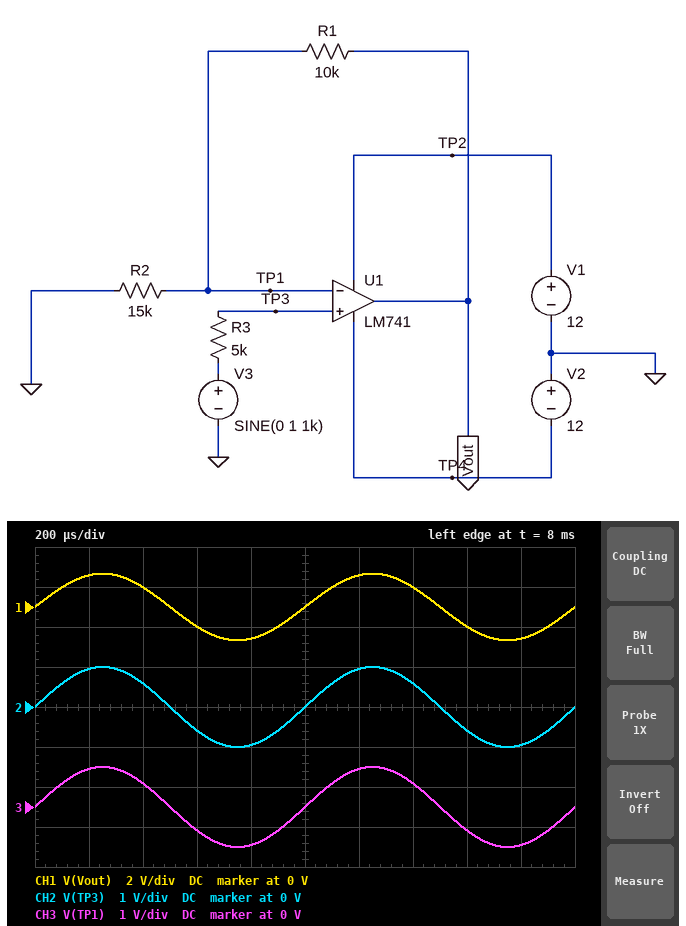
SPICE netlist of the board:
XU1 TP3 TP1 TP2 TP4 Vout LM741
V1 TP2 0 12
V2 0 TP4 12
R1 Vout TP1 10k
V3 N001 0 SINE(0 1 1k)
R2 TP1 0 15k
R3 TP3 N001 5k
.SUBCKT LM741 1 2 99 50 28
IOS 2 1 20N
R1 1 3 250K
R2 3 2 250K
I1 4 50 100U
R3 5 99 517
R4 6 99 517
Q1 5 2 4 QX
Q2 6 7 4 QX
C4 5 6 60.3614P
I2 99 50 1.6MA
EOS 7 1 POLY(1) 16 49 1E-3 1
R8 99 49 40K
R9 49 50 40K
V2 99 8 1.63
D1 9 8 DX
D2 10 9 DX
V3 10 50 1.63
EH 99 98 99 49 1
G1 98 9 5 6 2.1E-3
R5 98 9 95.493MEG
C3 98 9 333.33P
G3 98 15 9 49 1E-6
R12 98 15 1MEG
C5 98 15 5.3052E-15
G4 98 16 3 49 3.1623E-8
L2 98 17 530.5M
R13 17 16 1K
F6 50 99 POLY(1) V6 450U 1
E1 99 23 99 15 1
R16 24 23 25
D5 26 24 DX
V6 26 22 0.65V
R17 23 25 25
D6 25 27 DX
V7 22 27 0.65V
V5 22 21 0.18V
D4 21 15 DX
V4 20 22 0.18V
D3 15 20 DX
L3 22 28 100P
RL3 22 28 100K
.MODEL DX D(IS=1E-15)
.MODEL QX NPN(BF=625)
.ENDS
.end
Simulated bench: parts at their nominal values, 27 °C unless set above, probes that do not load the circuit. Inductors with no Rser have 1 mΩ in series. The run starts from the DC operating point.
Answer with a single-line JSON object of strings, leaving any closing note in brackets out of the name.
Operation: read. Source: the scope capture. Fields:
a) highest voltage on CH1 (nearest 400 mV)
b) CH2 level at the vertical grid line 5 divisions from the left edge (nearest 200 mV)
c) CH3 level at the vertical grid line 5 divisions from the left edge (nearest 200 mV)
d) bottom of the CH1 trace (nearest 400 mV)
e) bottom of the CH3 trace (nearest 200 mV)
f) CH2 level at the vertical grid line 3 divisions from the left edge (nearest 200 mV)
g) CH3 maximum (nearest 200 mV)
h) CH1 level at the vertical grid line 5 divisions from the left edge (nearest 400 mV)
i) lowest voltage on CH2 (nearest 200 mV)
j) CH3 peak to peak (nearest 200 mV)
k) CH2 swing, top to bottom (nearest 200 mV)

{"highest voltage on CH1": "1.6 V", "CH2 level at the vertical grid line 5 divisions from the left edge": "0 V", "CH3 level at the vertical grid line 5 divisions from the left edge": "0 V", "bottom of the CH1 trace": "-1.6 V", "bottom of the CH3 trace": "-1.0 V", "CH2 level at the vertical grid line 3 divisions from the left edge": "-600 mV", "CH3 maximum": "1.0 V", "CH1 level at the vertical grid line 5 divisions from the left edge": "0 V", "lowest voltage on CH2": "-1.0 V", "CH3 peak to peak": "2.0 V", "CH2 swing, top to bottom": "2.0 V"}
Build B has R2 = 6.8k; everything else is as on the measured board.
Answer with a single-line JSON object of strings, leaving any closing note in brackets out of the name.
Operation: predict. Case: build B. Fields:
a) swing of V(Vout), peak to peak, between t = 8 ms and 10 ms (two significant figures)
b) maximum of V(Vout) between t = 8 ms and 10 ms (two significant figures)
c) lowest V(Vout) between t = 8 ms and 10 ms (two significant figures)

{"swing of V(Vout), peak to peak, between t = 8 ms and 10 ms": "4.9 V", "maximum of V(Vout) between t = 8 ms and 10 ms": "2.5 V", "lowest V(Vout) between t = 8 ms and 10 ms": "-2.5 V"}
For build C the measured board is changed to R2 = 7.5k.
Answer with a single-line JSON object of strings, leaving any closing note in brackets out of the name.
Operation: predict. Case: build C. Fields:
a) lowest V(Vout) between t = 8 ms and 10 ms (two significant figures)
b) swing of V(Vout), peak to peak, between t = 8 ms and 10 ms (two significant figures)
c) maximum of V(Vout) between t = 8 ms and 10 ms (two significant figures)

{"lowest V(Vout) between t = 8 ms and 10 ms": "-2.3 V", "swing of V(Vout), peak to peak, between t = 8 ms and 10 ms": "4.7 V", "maximum of V(Vout) between t = 8 ms and 10 ms": "2.3 V"}
